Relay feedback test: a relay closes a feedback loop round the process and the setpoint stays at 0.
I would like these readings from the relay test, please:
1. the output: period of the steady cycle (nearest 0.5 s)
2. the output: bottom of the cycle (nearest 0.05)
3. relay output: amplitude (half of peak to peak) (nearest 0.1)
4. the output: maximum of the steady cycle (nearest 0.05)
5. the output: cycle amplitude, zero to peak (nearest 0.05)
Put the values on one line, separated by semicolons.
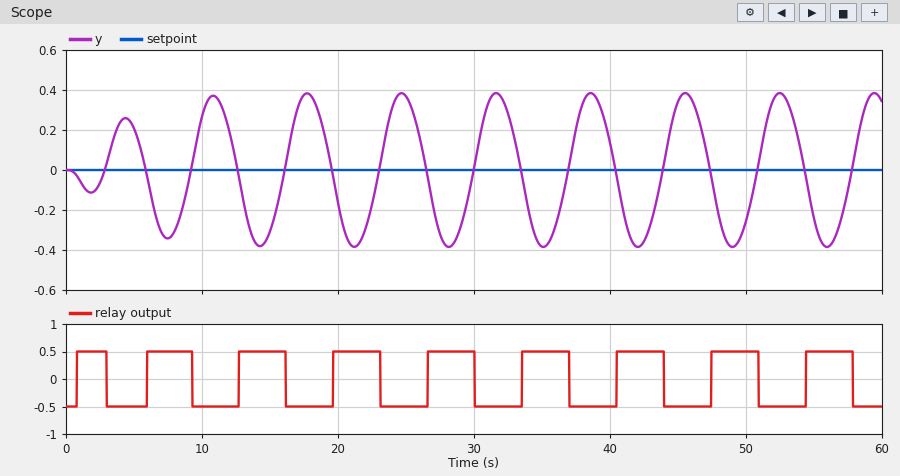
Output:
7.0 s; -0.40; 0.5; 0.40; 0.40
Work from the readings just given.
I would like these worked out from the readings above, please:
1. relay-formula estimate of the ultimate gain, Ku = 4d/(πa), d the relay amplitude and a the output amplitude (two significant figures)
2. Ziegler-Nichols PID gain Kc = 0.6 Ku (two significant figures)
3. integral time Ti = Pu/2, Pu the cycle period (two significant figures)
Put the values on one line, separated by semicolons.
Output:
1.6; 0.96; 3.5 s
